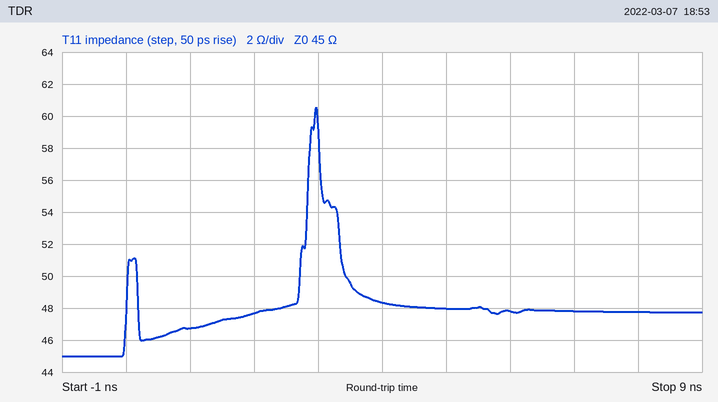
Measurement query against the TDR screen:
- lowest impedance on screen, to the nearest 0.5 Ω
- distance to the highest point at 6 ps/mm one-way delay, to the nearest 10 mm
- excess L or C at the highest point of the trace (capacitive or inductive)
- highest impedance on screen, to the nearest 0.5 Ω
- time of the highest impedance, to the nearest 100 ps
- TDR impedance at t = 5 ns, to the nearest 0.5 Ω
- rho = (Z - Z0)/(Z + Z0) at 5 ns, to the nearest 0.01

45.0 Ω
250 mm
inductive
60.5 Ω
3.0 ns
48.0 Ω
+0.03
